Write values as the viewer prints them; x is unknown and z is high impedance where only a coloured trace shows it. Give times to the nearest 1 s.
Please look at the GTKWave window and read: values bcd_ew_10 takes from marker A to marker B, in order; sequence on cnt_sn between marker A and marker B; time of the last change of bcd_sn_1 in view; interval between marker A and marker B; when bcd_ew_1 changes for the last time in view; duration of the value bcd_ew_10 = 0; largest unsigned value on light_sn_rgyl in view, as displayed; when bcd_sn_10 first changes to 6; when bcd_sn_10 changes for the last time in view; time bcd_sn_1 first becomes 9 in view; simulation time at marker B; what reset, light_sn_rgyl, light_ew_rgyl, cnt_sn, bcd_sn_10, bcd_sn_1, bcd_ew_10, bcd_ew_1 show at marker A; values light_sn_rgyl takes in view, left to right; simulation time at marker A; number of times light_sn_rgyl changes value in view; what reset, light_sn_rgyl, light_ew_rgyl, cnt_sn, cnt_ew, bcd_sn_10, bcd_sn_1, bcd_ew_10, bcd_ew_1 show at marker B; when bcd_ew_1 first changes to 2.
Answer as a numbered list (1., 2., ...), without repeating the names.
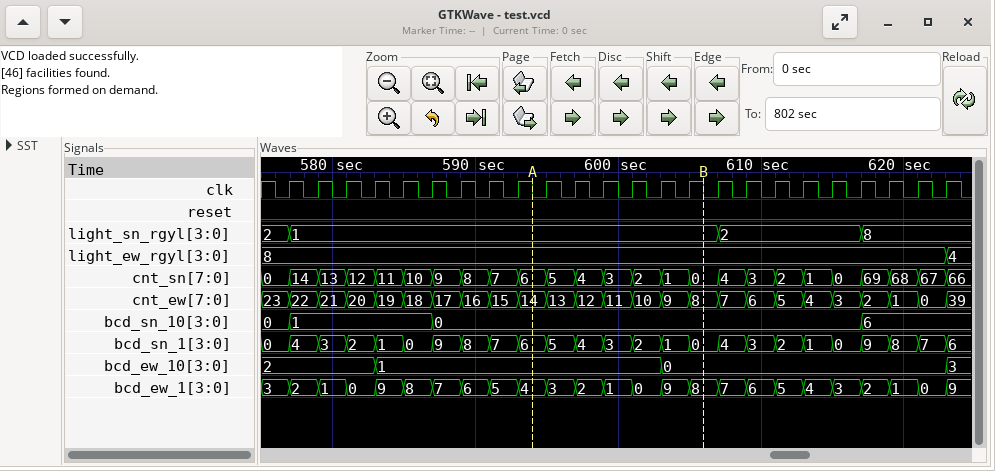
1. 1, 0
2. 6, 5, 4, 3, 2, 1, 0
3. 623 s
4. 12 s
5. 623 s
6. 20 s
7. 8
8. 617 s
9. 617 s
10. 587 s
11. 606 s
12. reset=0, light_sn_rgyl=1, light_ew_rgyl=8, cnt_sn=6, bcd_sn_10=0, bcd_sn_1=6, bcd_ew_10=1, bcd_ew_1=4
13. 2, 1, 2, 8
14. 594 s
15. 3
16. reset=0, light_sn_rgyl=1, light_ew_rgyl=8, cnt_sn=0, cnt_ew=8, bcd_sn_10=0, bcd_sn_1=0, bcd_ew_10=0, bcd_ew_1=8
17. 577 s
